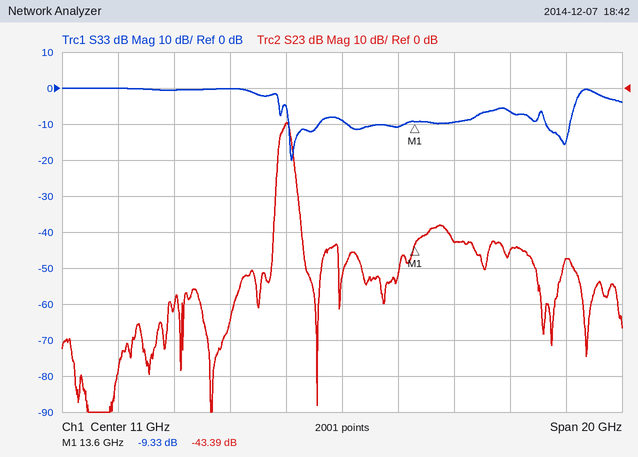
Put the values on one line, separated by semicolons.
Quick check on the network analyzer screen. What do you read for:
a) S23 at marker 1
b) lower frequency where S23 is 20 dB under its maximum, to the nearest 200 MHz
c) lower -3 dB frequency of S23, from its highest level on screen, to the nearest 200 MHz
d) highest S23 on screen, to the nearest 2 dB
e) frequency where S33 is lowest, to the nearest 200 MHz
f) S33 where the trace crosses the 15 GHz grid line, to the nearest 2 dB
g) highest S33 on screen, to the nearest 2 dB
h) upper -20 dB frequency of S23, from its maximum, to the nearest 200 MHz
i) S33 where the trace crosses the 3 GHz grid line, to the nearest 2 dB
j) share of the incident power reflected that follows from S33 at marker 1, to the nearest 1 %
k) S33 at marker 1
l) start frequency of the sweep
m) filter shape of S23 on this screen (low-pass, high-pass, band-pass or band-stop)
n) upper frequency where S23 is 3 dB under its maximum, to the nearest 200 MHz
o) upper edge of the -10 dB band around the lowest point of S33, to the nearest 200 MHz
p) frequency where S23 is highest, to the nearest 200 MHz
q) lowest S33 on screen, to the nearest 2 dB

-43.39 dB; 8.6 GHz; 8.8 GHz; -10 dB; 9.2 GHz; -10 dB; 0 dB; 9.4 GHz; 0 dB; 12 %; -9.33 dB; 1 GHz; band-pass; 9.2 GHz; 10.2 GHz; 9.0 GHz; -20 dB
